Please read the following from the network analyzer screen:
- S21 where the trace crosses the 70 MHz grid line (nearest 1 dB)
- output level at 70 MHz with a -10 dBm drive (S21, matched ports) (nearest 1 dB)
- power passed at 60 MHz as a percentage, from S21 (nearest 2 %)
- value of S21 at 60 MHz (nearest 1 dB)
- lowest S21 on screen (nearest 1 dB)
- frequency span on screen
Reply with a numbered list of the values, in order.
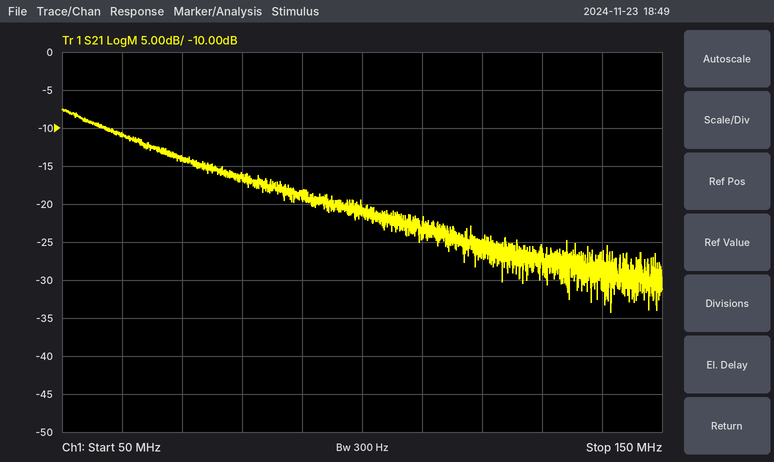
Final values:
1. -14 dB
2. -24 dBm
3. 8 %
4. -11 dB
5. -34 dB
6. 100 MHz
